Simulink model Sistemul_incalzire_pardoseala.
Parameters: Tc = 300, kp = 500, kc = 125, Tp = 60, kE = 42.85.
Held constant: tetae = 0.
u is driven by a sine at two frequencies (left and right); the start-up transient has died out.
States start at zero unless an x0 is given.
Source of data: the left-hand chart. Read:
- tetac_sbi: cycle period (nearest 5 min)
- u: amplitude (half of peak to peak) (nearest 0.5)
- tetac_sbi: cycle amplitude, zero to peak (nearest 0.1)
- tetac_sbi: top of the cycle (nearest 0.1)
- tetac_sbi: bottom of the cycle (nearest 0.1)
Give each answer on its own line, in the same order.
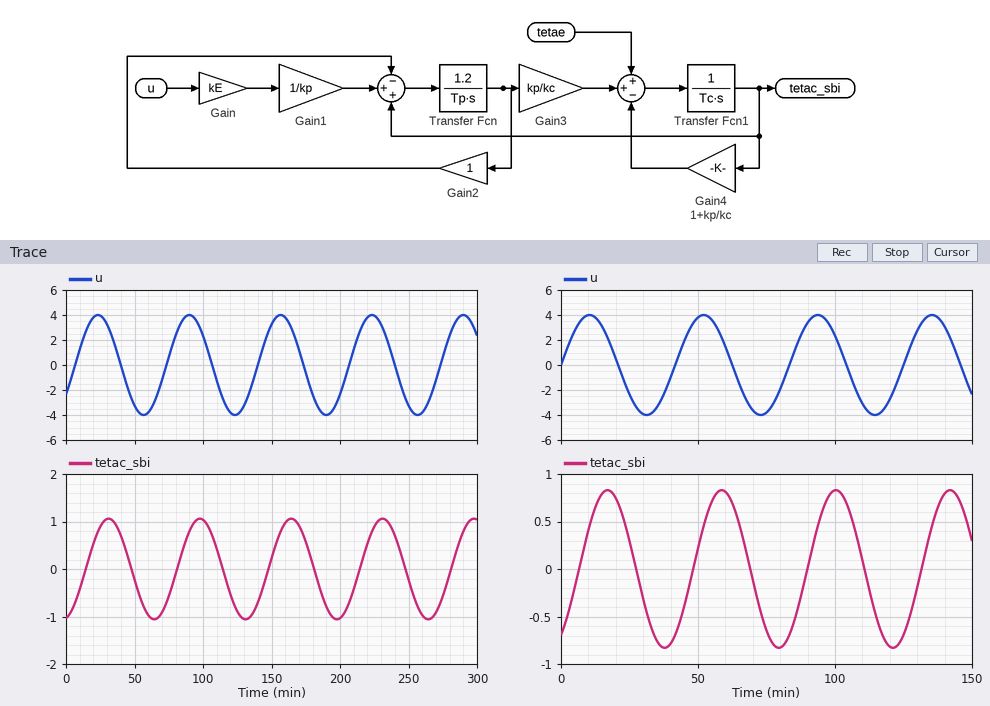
65 min
4.0
1.1
1.1
-1.1
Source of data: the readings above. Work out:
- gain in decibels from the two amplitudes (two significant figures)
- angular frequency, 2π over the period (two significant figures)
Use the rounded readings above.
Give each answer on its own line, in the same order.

-11 dB
0.097 rad/min
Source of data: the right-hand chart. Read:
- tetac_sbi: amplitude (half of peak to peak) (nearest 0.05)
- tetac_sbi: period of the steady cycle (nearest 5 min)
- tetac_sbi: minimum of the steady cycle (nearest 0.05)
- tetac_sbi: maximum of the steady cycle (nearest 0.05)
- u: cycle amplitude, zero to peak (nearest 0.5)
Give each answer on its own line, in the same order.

0.85
40 min
-0.85
0.85
4.0
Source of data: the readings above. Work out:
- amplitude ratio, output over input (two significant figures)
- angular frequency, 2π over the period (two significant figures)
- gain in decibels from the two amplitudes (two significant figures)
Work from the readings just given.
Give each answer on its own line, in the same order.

0.21
0.16 rad/min
-13 dB
